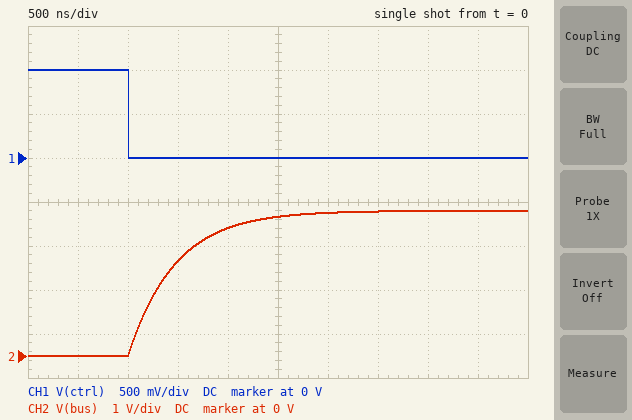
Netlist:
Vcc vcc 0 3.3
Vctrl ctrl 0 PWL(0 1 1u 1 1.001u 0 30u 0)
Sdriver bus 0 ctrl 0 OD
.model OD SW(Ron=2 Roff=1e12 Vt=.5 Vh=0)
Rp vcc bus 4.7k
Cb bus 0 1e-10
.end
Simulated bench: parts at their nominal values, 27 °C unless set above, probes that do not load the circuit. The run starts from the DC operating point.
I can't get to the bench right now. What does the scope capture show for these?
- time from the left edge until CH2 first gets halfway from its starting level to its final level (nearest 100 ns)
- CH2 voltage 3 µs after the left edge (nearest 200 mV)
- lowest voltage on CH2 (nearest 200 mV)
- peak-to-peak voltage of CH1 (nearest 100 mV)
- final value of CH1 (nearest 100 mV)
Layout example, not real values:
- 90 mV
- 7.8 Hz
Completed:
- 1.3 µs
- 3.2 V
- 0 V
- 1.0 V
- 0 V
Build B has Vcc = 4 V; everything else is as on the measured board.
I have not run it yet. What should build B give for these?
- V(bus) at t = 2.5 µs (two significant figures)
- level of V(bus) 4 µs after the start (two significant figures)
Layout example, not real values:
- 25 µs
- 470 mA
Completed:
- 3.8 V
- 4.0 V
